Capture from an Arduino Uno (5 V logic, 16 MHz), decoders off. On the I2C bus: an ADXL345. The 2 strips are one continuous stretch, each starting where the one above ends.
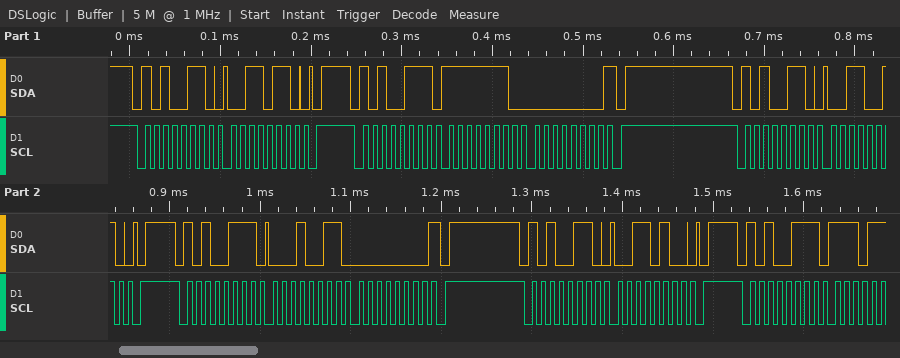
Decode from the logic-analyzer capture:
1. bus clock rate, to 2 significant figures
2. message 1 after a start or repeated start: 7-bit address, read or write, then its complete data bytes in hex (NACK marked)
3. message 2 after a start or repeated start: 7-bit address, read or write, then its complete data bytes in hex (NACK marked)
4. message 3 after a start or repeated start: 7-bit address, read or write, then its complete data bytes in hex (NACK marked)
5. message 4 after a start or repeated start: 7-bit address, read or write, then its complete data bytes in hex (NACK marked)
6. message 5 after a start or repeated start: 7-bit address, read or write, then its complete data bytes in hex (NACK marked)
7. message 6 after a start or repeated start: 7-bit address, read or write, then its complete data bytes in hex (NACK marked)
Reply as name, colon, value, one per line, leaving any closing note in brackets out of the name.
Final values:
bus clock rate, to 2 significant figures: 100 kHz
message 1 after a start or repeated start: 7-bit address, read or write, then its complete data bytes in hex: 0x53 write: 36
message 2 after a start or repeated start: 7-bit address, read or write, then its complete data bytes in hex: 0x53 read: FE 00 NACK
message 3 after a start or repeated start: 7-bit address, read or write, then its complete data bytes in hex: 0x53 write: 32
message 4 after a start or repeated start: 7-bit address, read or write, then its complete data bytes in hex: 0x53 read: 13 00 NACK
message 5 after a start or repeated start: 7-bit address, read or write, then its complete data bytes in hex: 0x53 write: 34
message 6 after a start or repeated start: 7-bit address, read or write, then its complete data bytes in hex: 0x53 read
